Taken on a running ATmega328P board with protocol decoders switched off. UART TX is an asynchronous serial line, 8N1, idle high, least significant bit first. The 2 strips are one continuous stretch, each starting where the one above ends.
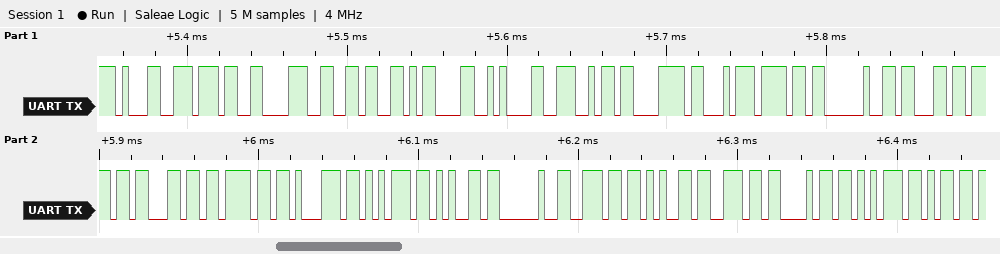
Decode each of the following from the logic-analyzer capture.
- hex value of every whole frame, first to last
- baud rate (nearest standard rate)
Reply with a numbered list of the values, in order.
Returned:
1. 31 37 38 36 0D 0A 4E C3 A3 6F 20 63 6F 6C 6F 71 75 65 20 6E 65 6E 68 75 6D
2. 250000 baud
